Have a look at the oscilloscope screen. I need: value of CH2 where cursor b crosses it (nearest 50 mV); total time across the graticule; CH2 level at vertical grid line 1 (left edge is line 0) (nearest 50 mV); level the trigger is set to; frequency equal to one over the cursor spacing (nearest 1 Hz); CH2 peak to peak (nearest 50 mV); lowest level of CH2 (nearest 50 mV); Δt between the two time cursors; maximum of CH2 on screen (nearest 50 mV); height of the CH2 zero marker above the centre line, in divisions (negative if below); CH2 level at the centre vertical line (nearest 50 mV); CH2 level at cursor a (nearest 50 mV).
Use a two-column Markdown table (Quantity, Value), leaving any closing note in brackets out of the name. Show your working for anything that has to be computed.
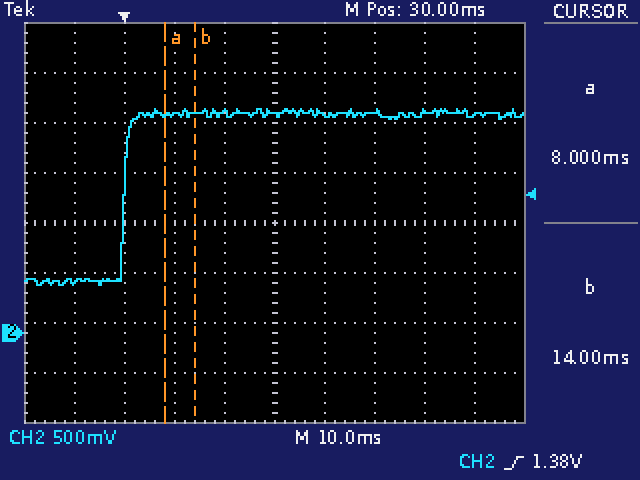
| Quantity | Value |
|---|---|
| value of CH2 where cursor b crosses it | 2.20 V |
| total time across the graticule | 100 ms |
| CH2 level at vertical grid line 1 (left edge is line 0) | 500 mV |
| level the trigger is set to | 1.38 V |
| frequency equal to one over the cursor spacing | 1 / 6 ms ≈ 167 Hz |
| CH2 peak to peak | 2.25 V − (500 mV) = 1.75 V |
| lowest level of CH2 | 500 mV |
| Δt between the two time cursors | 14 ms − (8 ms) = 6 ms |
| maximum of CH2 on screen | 2.25 V |
| height of the CH2 zero marker above the centre line, in divisions | -2.2 div |
| CH2 level at the centre vertical line | 2.20 V |
| CH2 level at cursor a | 2.20 V |
